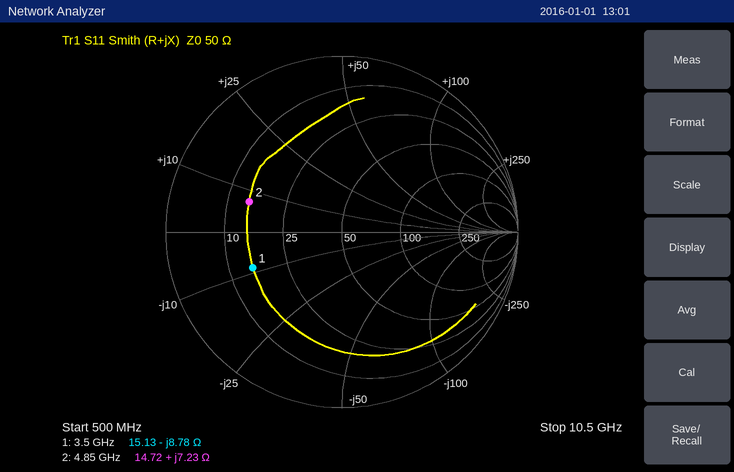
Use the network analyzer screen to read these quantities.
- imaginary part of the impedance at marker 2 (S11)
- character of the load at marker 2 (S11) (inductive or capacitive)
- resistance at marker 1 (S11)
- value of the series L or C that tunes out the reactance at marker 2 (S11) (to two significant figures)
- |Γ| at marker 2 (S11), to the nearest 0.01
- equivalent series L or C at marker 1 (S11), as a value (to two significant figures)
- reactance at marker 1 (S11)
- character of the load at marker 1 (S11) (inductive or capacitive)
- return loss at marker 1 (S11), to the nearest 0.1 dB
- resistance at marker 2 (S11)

+7.23 Ω
inductive
15.13 Ω
4.5 pF
0.55
5.2 pF
-8.78 Ω
capacitive
5.2 dB
14.72 Ω
